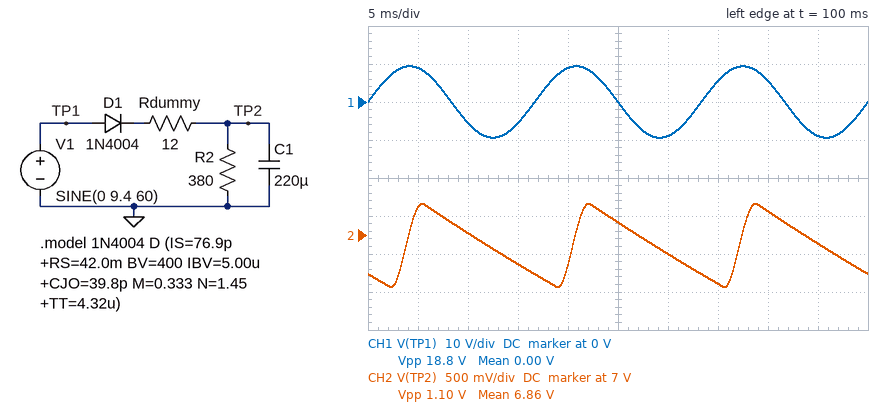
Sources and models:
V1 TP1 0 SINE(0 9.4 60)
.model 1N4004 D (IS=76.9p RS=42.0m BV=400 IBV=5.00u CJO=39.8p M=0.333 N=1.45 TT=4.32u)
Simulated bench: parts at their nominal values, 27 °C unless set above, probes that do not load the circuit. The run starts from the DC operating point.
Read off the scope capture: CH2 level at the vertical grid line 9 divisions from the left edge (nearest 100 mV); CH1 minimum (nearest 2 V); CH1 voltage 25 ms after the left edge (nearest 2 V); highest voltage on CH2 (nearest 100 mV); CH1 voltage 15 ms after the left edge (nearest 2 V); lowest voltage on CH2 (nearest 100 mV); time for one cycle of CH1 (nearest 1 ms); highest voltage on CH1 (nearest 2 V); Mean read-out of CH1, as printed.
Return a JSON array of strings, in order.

["6.9 V", "-10 V", "0 V", "7.4 V", "-6 V", "6.3 V", "17 ms", "10 V", "0.00 V"]
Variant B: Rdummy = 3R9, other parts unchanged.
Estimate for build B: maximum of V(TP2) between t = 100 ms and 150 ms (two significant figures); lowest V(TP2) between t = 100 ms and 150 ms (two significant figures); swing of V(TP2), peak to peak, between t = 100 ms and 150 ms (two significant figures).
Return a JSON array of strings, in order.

["8.2 V", "6.9 V", "1.3 V"]
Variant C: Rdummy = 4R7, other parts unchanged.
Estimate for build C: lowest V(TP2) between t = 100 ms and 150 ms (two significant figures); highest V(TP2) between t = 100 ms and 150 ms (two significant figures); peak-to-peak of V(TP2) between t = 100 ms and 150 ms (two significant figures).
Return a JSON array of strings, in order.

["6.9 V", "8.1 V", "1.3 V"]
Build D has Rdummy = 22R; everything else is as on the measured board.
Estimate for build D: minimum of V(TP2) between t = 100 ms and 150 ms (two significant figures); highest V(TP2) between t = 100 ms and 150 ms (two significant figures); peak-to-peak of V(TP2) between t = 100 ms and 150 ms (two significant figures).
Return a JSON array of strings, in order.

["5.7 V", "6.7 V", "970 mV"]
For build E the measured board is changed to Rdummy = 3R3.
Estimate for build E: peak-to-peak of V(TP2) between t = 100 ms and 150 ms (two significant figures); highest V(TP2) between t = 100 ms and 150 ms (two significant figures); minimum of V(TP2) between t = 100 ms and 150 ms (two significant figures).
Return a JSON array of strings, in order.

["1.3 V", "8.3 V", "7.0 V"]
